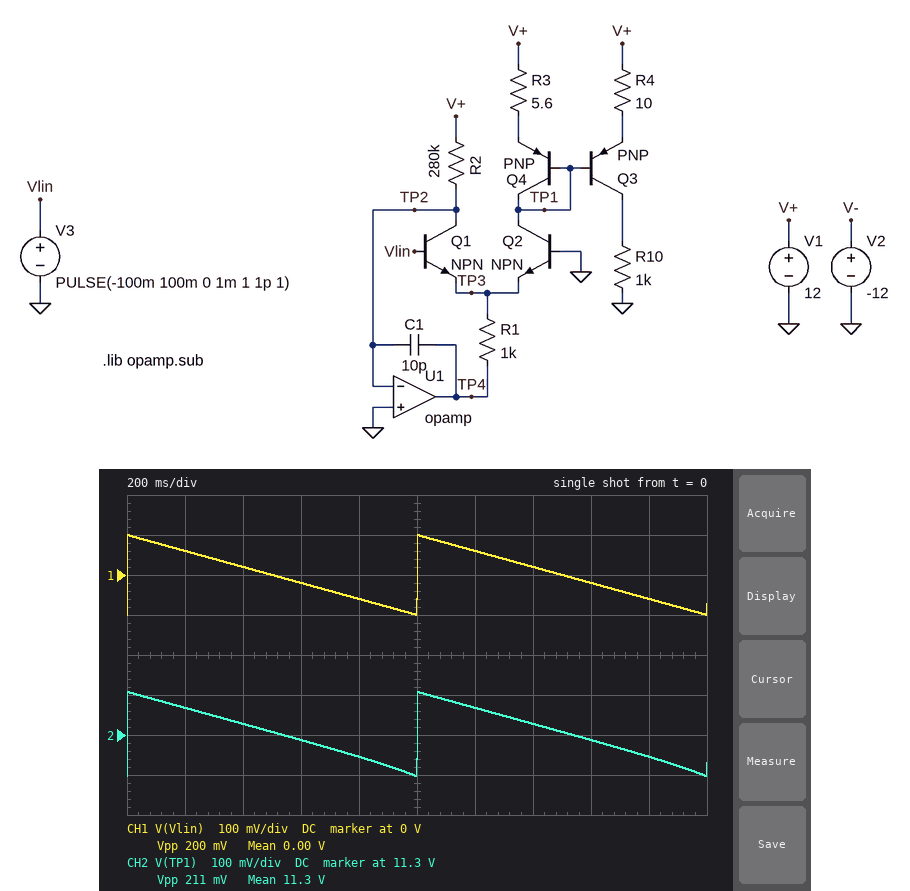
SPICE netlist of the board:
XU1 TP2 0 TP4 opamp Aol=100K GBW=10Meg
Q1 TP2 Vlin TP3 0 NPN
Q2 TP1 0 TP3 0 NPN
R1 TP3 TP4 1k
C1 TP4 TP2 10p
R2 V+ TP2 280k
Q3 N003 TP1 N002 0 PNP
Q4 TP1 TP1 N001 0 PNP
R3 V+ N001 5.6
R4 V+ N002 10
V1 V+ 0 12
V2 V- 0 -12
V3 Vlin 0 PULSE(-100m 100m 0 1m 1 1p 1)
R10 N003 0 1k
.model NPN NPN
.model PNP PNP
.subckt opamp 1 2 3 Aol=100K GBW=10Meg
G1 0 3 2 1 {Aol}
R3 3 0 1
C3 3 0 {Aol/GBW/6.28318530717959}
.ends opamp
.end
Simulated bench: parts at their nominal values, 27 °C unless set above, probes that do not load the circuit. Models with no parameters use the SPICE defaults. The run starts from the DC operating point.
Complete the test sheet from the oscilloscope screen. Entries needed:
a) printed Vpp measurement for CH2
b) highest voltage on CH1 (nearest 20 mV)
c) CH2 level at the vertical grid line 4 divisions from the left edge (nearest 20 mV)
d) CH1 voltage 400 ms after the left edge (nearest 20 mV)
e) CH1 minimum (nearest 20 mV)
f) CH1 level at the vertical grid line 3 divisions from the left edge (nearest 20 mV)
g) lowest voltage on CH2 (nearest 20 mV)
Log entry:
211 mV
100 mV
11.24 V
20 mV
-100 mV
-20 mV
11.20 V
